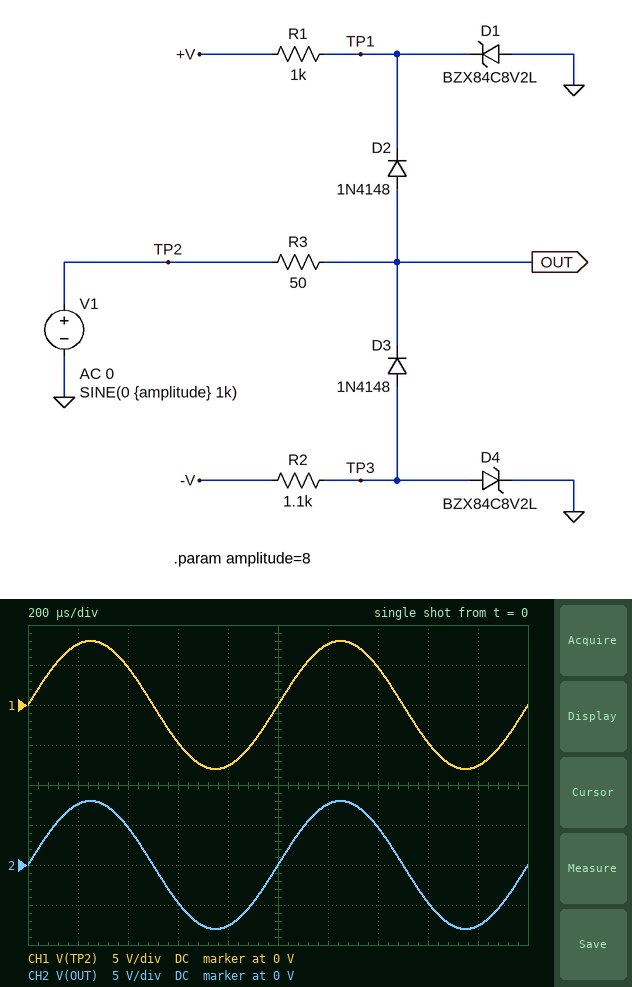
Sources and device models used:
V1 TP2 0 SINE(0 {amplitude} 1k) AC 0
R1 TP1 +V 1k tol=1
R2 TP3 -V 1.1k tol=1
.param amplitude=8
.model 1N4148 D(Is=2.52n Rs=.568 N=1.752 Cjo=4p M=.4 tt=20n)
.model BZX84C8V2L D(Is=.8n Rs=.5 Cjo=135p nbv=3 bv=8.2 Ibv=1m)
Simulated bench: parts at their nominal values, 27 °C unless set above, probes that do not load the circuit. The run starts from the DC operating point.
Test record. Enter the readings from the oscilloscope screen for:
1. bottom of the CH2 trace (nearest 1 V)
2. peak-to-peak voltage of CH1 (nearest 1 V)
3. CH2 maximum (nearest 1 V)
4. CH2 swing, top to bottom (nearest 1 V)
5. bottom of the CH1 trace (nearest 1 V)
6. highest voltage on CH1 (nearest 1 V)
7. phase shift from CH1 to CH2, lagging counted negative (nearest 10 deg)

-8 V
16 V
8 V
16 V
-8 V
8 V
0 deg
